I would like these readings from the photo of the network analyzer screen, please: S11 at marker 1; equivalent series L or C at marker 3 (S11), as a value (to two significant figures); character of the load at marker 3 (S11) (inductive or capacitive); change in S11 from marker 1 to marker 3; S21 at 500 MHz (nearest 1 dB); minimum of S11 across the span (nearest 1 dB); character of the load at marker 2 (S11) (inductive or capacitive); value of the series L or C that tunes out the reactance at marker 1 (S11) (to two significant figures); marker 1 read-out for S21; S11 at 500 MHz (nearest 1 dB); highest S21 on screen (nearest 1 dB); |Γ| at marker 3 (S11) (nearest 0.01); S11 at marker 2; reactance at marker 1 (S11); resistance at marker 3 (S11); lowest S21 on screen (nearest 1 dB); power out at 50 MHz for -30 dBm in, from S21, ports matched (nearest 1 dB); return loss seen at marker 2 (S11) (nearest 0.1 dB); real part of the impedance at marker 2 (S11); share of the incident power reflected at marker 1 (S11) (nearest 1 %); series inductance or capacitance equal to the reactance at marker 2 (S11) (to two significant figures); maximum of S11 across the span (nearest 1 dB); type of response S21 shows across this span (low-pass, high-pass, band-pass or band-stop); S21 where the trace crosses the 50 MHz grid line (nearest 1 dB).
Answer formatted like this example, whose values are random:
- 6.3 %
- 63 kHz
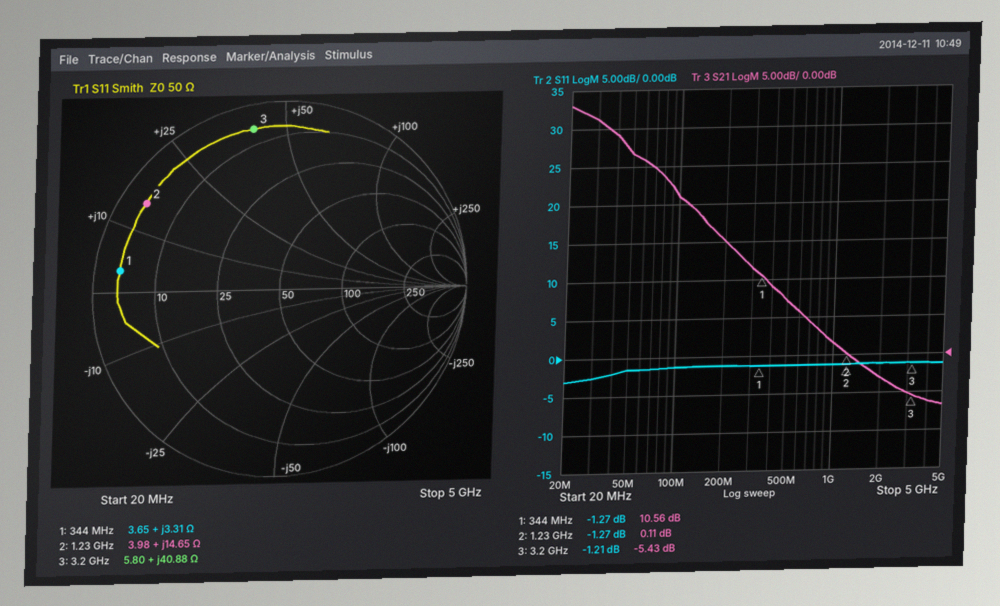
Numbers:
- -1.27 dB
- 2.0 nH
- inductive
- 0.06 dB
- 7 dB
- -3 dB
- inductive
- 140 pF
- 10.56 dB
- -1 dB
- 33 dB
- 0.87
- -1.27 dB
- +3.31 Ω
- 5.80 Ω
- -7 dB
- -3 dBm
- 1.3 dB
- 3.98 Ω
- 75 %
- 1.9 nH
- -1 dB
- low-pass
- 27 dB
